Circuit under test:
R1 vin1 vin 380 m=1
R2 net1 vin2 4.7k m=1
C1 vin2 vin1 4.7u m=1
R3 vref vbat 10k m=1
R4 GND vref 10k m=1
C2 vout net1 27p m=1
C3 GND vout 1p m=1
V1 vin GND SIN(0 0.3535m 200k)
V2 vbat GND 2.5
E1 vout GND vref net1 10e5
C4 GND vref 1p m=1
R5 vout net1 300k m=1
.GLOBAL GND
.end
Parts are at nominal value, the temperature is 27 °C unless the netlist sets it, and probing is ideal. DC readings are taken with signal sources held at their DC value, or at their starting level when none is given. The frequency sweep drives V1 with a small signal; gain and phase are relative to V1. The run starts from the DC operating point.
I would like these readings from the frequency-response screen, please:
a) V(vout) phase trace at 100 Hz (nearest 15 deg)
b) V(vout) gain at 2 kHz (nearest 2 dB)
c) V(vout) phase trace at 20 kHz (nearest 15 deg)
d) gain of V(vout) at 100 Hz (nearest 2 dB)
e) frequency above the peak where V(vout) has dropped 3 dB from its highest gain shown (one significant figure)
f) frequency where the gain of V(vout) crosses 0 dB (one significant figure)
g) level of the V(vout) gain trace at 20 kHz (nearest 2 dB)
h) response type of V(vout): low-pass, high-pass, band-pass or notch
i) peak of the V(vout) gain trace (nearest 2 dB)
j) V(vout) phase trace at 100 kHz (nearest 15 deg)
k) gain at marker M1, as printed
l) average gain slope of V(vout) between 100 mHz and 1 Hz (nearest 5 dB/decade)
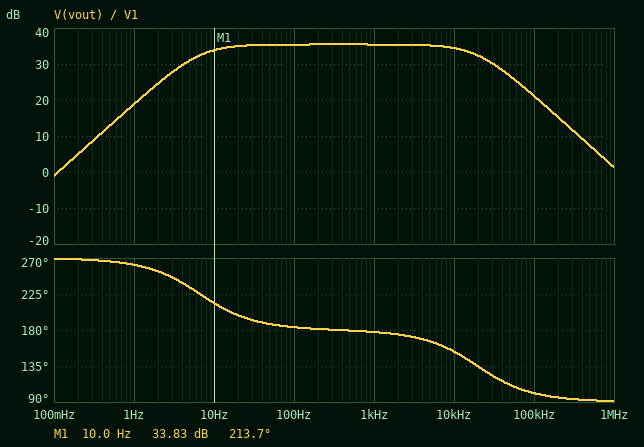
180 deg
36 dB
135 deg
36 dB
20 kHz
100 mHz
32 dB
band-pass
36 dB
105 deg
33.83 dB
20 dB/decade
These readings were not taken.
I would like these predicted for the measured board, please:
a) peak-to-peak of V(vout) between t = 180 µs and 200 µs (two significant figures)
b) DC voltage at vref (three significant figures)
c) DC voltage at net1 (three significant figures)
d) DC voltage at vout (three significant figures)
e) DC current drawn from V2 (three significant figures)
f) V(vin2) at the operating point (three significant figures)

4.1 mV
1.25 V
1.25 V
1.25 V
125 µA
1.25 V
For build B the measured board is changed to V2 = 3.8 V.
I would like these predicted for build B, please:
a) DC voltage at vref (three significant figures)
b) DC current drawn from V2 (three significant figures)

1.90 V
190 µA
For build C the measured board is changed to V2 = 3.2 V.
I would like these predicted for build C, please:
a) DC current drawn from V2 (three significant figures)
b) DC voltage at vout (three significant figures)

160 µA
1.60 V
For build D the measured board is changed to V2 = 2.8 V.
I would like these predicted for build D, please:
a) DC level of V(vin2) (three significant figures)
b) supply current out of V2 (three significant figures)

1.40 V
140 µA
